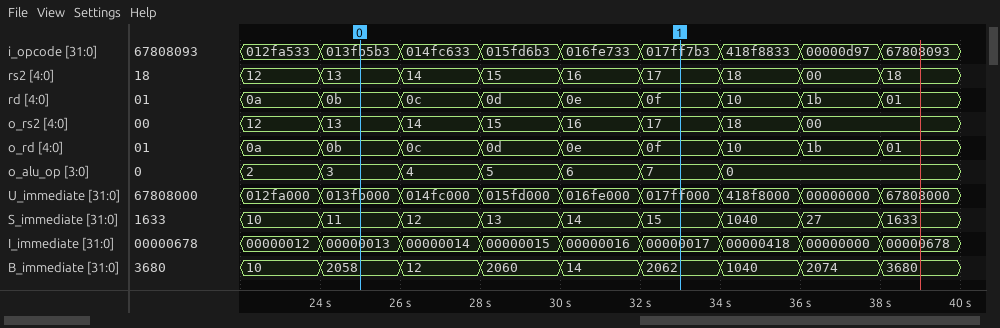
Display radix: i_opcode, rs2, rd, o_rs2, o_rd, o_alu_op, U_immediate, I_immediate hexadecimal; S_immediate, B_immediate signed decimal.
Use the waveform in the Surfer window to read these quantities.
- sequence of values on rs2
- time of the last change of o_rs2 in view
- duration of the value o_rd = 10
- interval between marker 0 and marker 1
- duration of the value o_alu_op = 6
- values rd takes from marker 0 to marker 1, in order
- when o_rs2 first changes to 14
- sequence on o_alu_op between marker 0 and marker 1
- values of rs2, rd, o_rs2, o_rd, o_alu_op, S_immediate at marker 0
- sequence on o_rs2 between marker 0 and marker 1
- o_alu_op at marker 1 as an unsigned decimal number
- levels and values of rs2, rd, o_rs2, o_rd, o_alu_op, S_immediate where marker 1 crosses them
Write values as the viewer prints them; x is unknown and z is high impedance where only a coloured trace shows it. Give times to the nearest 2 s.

12, 13, 14, 15, 16, 17, 18, 00, 18
36 s
2 s
8 s
2 s
0b, 0c, 0d, 0e, 0f
26 s
3, 4, 5, 6, 7
rs2=13, rd=0b, o_rs2=13, o_rd=0b, o_alu_op=3, S_immediate=11
13, 14, 15, 16, 17
7
rs2=17, rd=0f, o_rs2=17, o_rd=0f, o_alu_op=7, S_immediate=15
